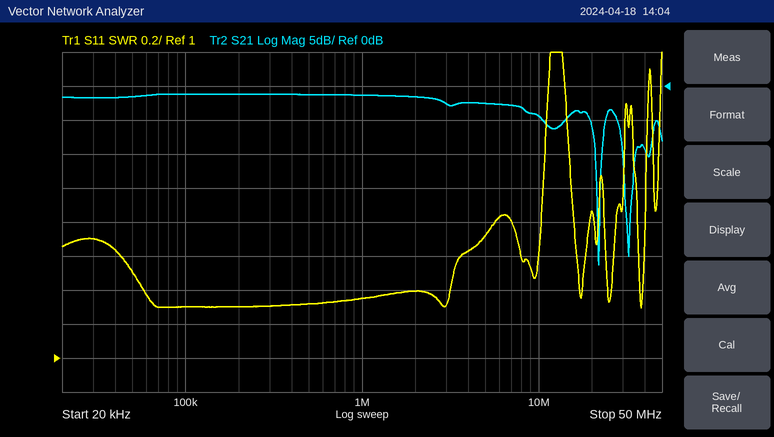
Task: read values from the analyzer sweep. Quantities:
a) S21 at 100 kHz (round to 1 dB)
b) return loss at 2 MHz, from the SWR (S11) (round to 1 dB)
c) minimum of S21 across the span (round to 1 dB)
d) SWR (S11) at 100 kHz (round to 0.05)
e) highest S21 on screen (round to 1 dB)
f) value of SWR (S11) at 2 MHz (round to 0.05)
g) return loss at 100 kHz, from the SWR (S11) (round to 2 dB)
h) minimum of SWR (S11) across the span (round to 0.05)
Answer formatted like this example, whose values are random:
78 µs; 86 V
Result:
-1 dB; 16 dB; -26 dB; 1.30; -1 dB; 1.40; 18 dB; 1.30
